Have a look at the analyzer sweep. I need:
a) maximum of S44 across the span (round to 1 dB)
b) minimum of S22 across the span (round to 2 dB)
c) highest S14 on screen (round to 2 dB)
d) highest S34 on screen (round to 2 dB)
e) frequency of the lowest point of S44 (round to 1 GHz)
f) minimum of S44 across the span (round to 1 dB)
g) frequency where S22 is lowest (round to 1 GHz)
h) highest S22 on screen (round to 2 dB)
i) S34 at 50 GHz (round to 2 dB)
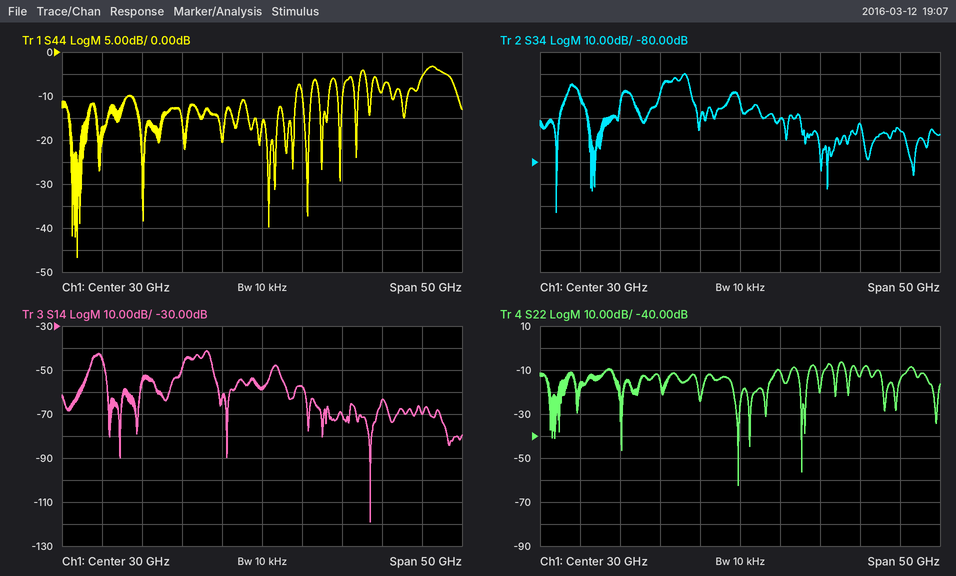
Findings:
-3 dB
-62 dB
-42 dB
-40 dB
7 GHz
-47 dB
30 GHz
-6 dB
-66 dB
